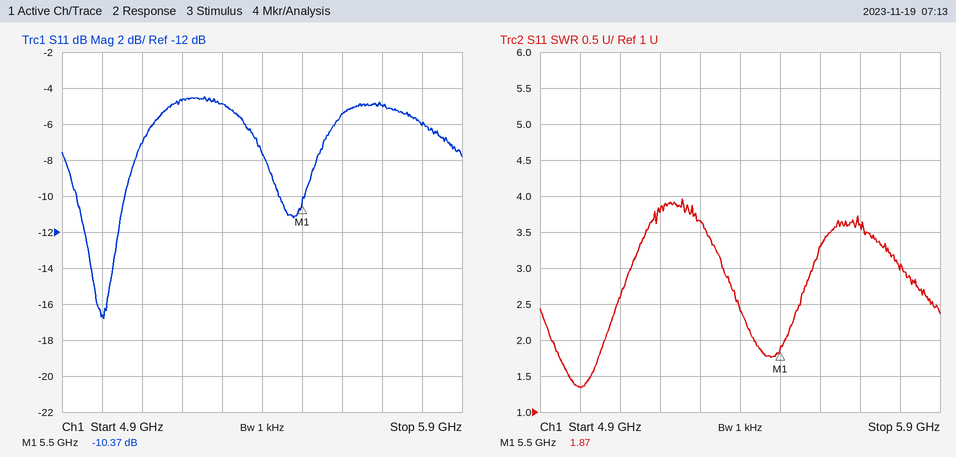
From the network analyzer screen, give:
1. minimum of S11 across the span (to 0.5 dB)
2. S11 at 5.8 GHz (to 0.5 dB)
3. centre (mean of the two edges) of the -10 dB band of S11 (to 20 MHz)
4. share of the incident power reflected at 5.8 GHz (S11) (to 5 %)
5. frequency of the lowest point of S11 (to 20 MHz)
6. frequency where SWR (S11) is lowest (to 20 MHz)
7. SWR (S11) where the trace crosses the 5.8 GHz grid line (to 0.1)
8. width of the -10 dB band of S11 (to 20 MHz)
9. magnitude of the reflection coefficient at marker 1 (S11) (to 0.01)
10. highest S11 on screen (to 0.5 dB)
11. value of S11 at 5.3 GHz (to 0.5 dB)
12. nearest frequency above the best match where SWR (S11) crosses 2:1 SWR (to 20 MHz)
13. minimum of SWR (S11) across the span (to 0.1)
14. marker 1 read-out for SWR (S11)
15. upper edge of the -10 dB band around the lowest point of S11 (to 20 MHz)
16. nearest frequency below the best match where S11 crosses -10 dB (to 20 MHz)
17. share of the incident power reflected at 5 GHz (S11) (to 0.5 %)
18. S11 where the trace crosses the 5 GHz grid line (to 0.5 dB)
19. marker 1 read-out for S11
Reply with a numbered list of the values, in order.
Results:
1. -17.0 dB
2. -6.0 dB
3. 5.00 GHz
4. 25 %
5. 5.00 GHz
6. 5.00 GHz
7. 3.0
8. 120 MHz
9. 0.30
10. -4.5 dB
11. -5.0 dB
12. 5.06 GHz
13. 1.3
14. 1.87
15. 5.06 GHz
16. 4.94 GHz
17. 2.0 %
18. -16.5 dB
19. -10.37 dB
